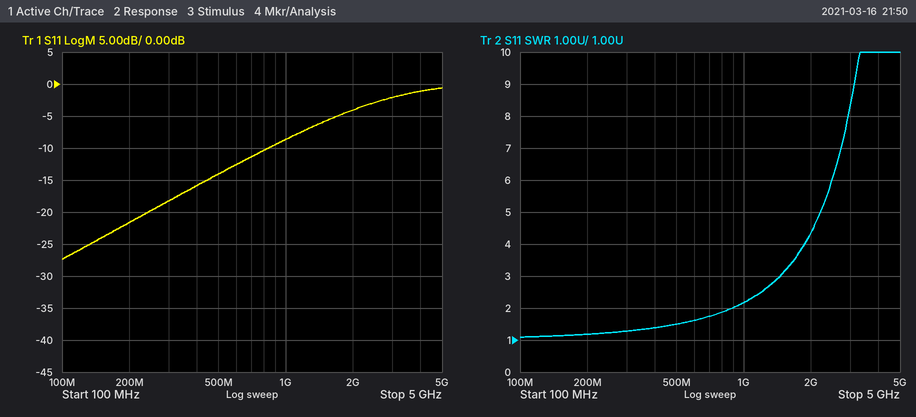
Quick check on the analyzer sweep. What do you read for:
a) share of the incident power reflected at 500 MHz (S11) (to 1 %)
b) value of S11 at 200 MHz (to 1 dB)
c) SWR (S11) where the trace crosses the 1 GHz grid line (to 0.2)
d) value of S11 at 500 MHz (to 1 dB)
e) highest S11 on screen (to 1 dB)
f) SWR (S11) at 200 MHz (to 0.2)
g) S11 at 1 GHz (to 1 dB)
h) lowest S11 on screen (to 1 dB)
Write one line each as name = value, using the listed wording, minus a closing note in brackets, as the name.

share of the incident power reflected at 500 MHz (S11) = 4 %
value of S11 at 200 MHz = -22 dB
SWR (S11) where the trace crosses the 1 GHz grid line = 2.2
value of S11 at 500 MHz = -14 dB
highest S11 on screen = -1 dB
SWR (S11) at 200 MHz = 1.2
S11 at 1 GHz = -9 dB
lowest S11 on screen = -27 dB
